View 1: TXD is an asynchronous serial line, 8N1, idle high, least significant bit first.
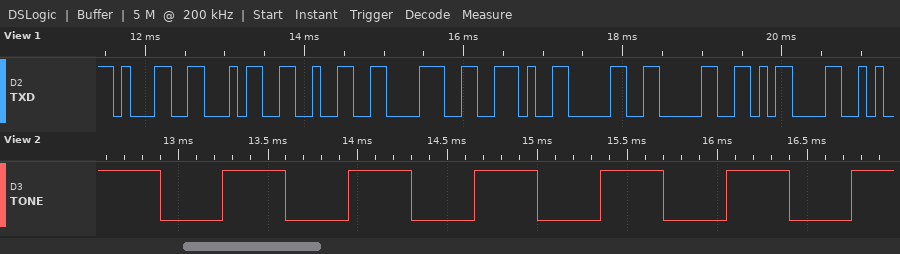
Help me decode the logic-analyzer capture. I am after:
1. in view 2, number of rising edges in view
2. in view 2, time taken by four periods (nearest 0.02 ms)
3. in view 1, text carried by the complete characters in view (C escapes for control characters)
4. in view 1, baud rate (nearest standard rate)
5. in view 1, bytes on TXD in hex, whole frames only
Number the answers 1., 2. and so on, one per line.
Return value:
1. 6
2. 2.80 ms
3. "1428.00\r"
4. 9600 baud
5. 31 34 32 38 2E 30 30 0D
